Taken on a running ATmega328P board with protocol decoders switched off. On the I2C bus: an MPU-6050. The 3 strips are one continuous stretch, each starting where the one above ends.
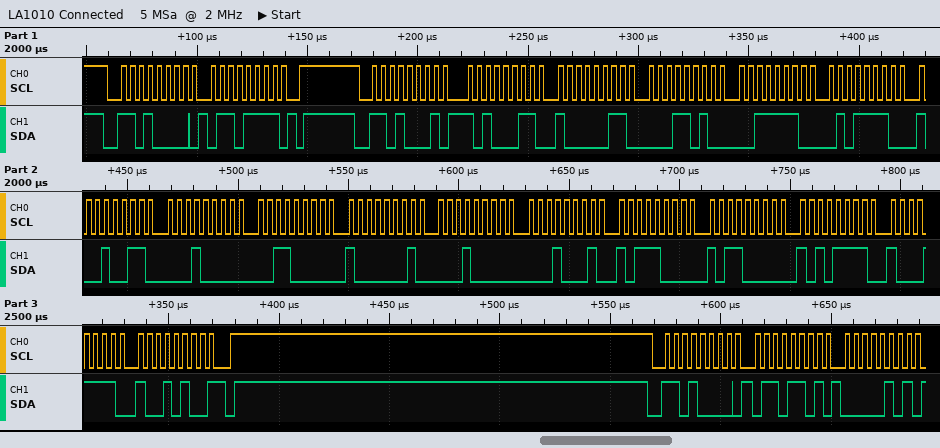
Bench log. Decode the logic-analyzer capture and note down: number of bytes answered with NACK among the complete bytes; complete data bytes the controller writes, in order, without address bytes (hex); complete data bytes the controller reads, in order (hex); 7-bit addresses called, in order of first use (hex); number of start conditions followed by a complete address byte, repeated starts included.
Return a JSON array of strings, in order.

["1", "6F 6D 05", "A3 83 1A 3E 5E 93 10 30 81 10 11 B8 B0 AF 8F 94", "0x68", "3"]
